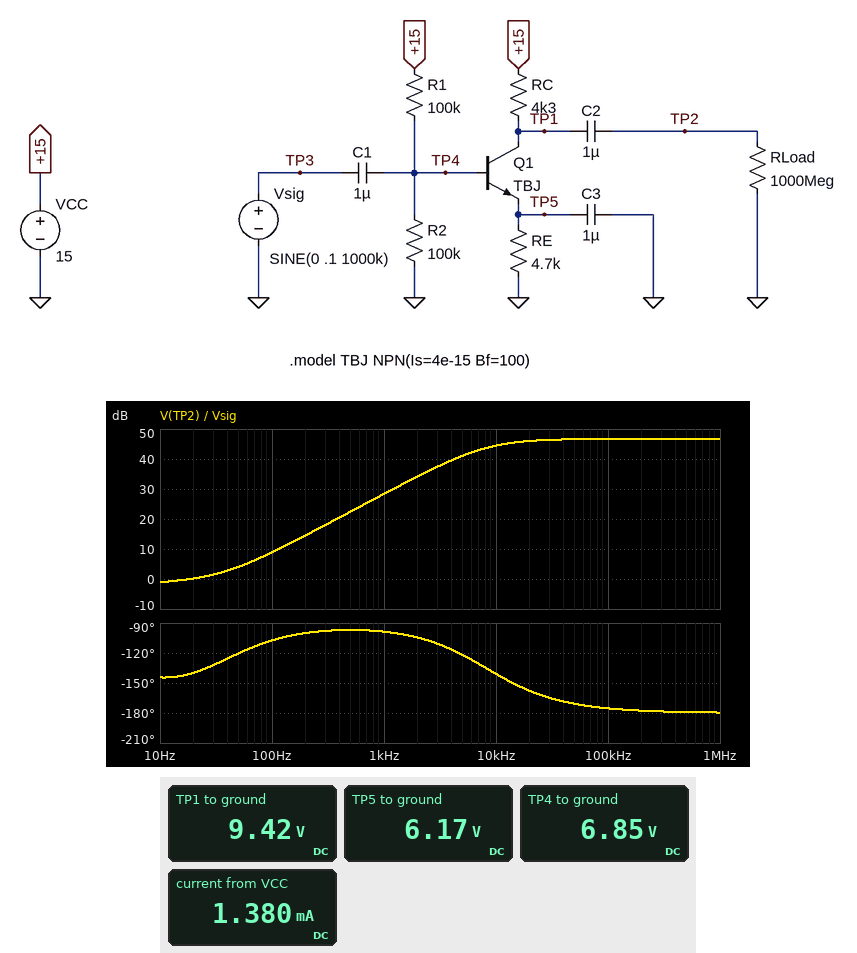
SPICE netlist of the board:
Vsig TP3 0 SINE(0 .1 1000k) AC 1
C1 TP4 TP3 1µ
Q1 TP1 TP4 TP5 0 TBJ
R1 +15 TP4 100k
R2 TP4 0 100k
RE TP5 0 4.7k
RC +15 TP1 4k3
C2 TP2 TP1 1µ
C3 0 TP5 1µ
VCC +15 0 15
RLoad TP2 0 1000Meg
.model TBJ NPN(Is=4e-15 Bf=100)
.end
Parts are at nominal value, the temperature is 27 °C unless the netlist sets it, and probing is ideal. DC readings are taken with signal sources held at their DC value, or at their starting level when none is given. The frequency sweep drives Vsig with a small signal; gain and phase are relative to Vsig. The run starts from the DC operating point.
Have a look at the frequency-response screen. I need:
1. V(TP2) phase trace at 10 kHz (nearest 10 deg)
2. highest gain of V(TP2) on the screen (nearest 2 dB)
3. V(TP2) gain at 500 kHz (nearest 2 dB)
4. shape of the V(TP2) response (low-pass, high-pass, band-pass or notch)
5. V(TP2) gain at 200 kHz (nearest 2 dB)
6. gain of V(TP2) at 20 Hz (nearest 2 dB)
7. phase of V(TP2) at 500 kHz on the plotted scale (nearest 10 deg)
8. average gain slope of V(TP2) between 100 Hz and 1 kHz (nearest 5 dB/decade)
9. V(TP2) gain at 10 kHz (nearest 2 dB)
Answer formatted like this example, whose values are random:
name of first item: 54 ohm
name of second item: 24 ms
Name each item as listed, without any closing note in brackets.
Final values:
V(TP2) phase trace at 10 kHz: -140 deg
highest gain of V(TP2) on the screen: 46 dB
V(TP2) gain at 500 kHz: 46 dB
shape of the V(TP2) response: high-pass
V(TP2) gain at 200 kHz: 46 dB
gain of V(TP2) at 20 Hz: 0 dB
phase of V(TP2) at 500 kHz on the plotted scale: -180 deg
average gain slope of V(TP2) between 100 Hz and 1 kHz: 20 dB/decade
V(TP2) gain at 10 kHz: 44 dB
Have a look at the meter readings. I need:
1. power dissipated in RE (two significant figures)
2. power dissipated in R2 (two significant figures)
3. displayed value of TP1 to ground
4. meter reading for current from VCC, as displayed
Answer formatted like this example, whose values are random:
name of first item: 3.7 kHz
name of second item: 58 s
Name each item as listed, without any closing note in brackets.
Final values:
power dissipated in RE: 8.1 mW
power dissipated in R2: 470 µW
displayed value of TP1 to ground: 9.42 V
meter reading for current from VCC, as displayed: 1.380 mA
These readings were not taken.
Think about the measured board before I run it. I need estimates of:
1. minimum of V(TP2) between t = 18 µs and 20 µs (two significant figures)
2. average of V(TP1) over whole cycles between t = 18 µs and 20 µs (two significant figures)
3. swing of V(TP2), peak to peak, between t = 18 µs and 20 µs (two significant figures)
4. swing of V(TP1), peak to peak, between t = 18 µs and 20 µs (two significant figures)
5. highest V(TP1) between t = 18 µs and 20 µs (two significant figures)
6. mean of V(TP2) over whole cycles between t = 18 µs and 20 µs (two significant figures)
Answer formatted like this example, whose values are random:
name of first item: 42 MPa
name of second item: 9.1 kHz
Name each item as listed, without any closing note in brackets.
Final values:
minimum of V(TP2) between t = 18 µs and 20 µs: -3.2 V
average of V(TP1) over whole cycles between t = 18 µs and 20 µs: 12 V
swing of V(TP2), peak to peak, between t = 18 µs and 20 µs: 8.8 V
swing of V(TP1), peak to peak, between t = 18 µs and 20 µs: 8.8 V
highest V(TP1) between t = 18 µs and 20 µs: 15 V
mean of V(TP2) over whole cycles between t = 18 µs and 20 µs: 2.2 V
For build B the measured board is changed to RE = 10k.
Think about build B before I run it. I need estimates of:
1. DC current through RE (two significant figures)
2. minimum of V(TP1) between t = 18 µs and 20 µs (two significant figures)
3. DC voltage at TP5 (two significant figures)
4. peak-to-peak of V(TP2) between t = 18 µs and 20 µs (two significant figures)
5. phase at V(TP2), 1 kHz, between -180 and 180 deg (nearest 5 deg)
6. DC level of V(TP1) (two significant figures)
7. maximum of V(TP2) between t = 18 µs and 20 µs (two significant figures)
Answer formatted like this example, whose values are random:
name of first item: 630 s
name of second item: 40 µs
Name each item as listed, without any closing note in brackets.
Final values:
DC current through RE: 650 µA
minimum of V(TP1) between t = 18 µs and 20 µs: 6.6 V
DC voltage at TP5: 6.5 V
peak-to-peak of V(TP2) between t = 18 µs and 20 µs: 8.4 V
phase at V(TP2), 1 kHz, between -180 and 180 deg: -105 deg
DC level of V(TP1): 12 V
maximum of V(TP2) between t = 18 µs and 20 µs: 2.8 V
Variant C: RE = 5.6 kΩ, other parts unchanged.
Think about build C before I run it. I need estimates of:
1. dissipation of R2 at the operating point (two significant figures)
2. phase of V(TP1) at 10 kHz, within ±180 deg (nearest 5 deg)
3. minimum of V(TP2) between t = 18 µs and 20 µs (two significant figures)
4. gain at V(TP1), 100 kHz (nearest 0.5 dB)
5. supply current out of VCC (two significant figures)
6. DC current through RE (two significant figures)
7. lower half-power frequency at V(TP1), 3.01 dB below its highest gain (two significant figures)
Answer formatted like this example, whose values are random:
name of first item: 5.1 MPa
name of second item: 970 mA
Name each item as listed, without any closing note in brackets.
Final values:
dissipation of R2 at the operating point: 480 µW
phase of V(TP1) at 10 kHz, within ±180 deg: -145 deg
minimum of V(TP2) between t = 18 µs and 20 µs: -3.9 V
gain at V(TP1), 100 kHz: 45.5 dB
supply current out of VCC: 1.2 mA
DC current through RE: 1.1 mA
lower half-power frequency at V(TP1), 3.01 dB below its highest gain: 7.0 kHz
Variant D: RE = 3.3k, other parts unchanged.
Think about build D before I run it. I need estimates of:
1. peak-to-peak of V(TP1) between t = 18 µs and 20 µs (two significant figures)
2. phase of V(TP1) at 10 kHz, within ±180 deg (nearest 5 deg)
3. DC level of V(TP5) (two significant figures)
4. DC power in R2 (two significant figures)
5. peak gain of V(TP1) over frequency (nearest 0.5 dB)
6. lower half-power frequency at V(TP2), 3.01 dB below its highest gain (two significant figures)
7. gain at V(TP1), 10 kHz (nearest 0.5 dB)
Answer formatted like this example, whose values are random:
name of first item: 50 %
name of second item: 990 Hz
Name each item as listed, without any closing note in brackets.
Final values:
peak-to-peak of V(TP1) between t = 18 µs and 20 µs: 9.0 V
phase of V(TP1) at 10 kHz, within ±180 deg: -130 deg
DC level of V(TP5): 5.9 V
DC power in R2: 440 µW
peak gain of V(TP1) over frequency: 49.5 dB
lower half-power frequency at V(TP2), 3.01 dB below its highest gain: 11 kHz
gain at V(TP1), 10 kHz: 46.0 dB
